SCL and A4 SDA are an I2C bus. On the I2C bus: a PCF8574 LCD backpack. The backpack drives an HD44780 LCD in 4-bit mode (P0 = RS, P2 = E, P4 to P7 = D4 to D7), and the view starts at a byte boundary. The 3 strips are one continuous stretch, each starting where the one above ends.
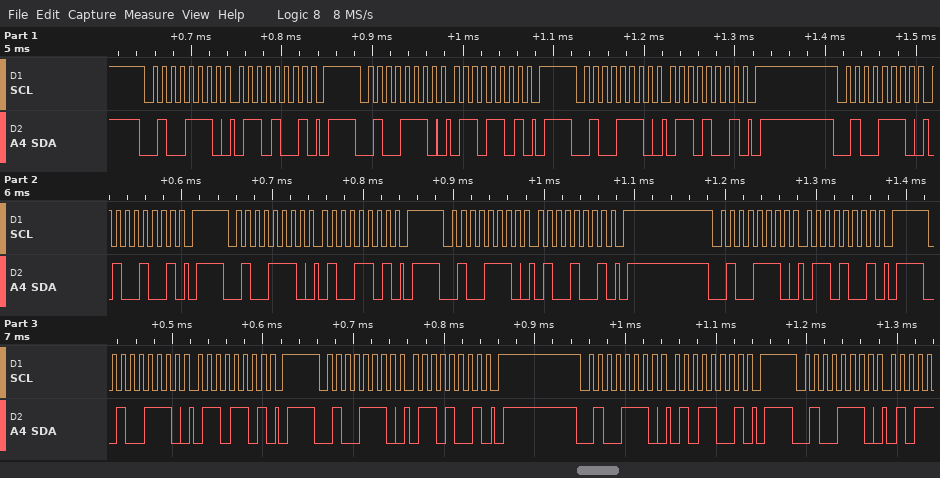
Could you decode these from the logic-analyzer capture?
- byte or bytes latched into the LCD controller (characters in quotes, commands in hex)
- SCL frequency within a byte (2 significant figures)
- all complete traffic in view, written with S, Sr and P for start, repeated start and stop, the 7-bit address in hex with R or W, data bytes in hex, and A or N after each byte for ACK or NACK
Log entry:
'd'
100 kHz
S 27W A 69 A P S 27W A 6D A P S 27W A 69 A P S 27W A 49 A P S 27W A 4D A P S 27W A 49 A P S 27W A 69 A P S 27W A 6D A P S 27W A 69 A P S 27W A 59 A P S 27W A
